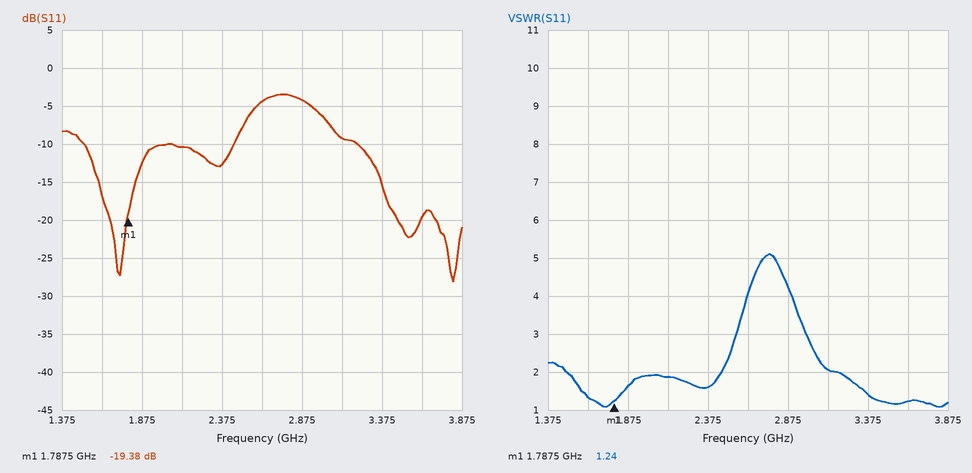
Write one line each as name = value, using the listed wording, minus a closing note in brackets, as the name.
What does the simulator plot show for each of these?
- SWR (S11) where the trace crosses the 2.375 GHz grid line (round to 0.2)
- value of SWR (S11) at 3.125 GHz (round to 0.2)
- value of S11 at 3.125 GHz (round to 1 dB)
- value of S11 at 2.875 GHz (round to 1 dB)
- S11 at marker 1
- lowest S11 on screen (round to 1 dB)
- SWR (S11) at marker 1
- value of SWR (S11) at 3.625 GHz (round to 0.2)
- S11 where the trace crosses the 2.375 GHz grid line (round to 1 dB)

SWR (S11) where the trace crosses the 2.375 GHz grid line = 1.6
value of SWR (S11) at 3.125 GHz = 2.0
value of S11 at 3.125 GHz = -9 dB
value of S11 at 2.875 GHz = -4 dB
S11 at marker 1 = -19.38 dB
lowest S11 on screen = -28 dB
SWR (S11) at marker 1 = 1.24
value of SWR (S11) at 3.625 GHz = 1.2
S11 where the trace crosses the 2.375 GHz grid line = -13 dB
